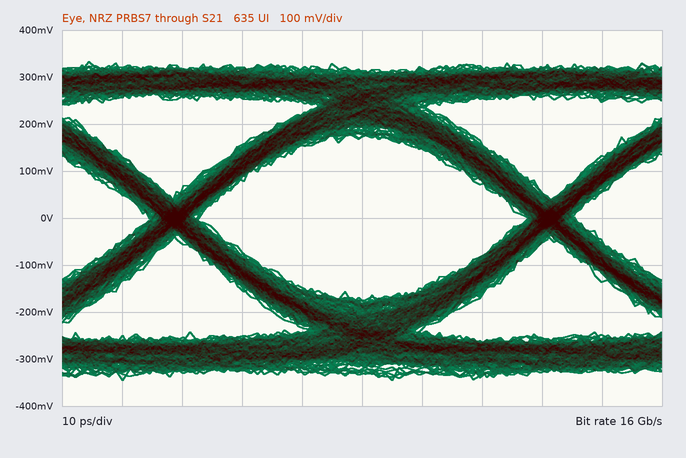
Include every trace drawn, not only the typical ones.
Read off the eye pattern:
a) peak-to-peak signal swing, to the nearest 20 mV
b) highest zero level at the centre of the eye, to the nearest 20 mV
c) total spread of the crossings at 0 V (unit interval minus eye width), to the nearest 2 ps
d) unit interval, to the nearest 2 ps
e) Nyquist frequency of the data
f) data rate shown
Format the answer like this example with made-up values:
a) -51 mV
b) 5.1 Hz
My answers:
a) 680 mV
b) -180 mV
c) 8 ps
d) 62 ps
e) 8 GHz
f) 16 Gb/s
